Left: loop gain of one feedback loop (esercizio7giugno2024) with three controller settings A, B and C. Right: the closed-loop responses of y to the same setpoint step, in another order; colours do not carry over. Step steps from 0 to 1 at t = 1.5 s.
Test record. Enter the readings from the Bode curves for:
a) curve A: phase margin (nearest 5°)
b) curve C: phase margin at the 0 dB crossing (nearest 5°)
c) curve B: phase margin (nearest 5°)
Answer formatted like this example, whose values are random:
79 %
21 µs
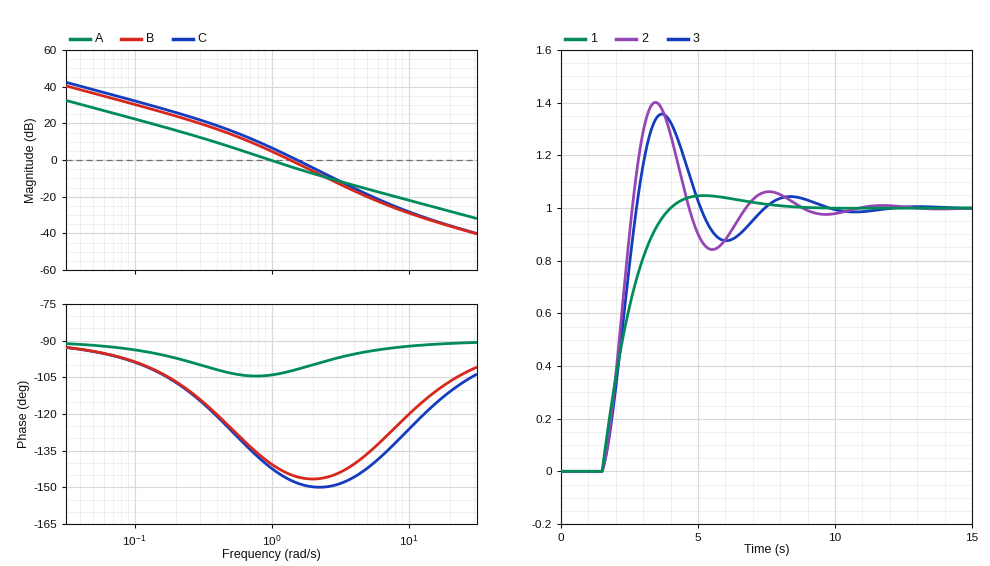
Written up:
75°
30°
35°
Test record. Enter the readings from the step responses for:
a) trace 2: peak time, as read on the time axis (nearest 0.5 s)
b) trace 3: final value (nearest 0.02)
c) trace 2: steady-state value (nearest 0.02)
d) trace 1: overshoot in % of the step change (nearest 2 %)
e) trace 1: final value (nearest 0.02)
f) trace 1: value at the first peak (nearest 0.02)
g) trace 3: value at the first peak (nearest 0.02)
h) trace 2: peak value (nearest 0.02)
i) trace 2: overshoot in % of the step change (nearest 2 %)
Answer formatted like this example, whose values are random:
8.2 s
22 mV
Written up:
3.5 s
1.00
1.00
4 %
1.00
1.04
1.36
1.40
40 %
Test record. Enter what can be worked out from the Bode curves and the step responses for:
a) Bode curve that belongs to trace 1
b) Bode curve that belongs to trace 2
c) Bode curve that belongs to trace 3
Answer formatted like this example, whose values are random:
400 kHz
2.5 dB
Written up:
A
C
B
